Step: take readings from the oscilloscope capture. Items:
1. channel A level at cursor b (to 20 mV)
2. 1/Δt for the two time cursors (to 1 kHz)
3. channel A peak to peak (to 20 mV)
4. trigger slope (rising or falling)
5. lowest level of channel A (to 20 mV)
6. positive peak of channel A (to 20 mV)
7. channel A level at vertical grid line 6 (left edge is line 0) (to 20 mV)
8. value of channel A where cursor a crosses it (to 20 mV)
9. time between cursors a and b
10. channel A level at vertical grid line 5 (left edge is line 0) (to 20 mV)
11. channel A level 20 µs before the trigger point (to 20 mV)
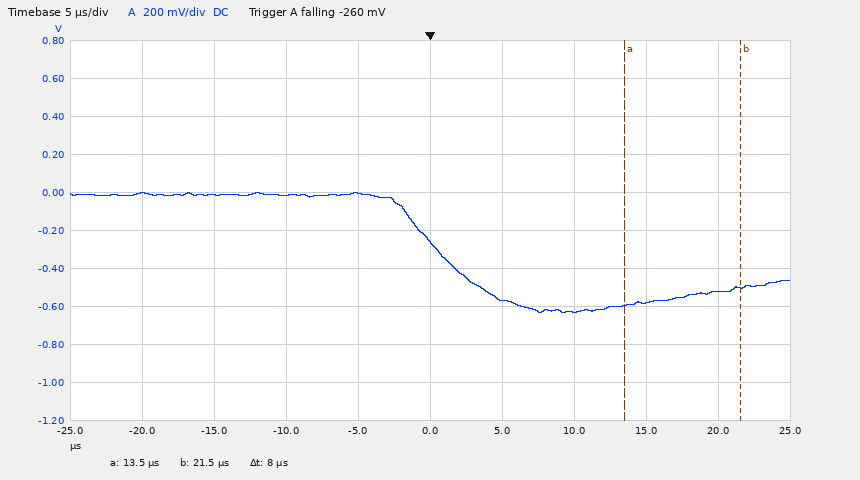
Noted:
-500 mV
125 kHz
640 mV
falling
-640 mV
0 mV
-560 mV
-600 mV
8 µs
-260 mV
0 mV
